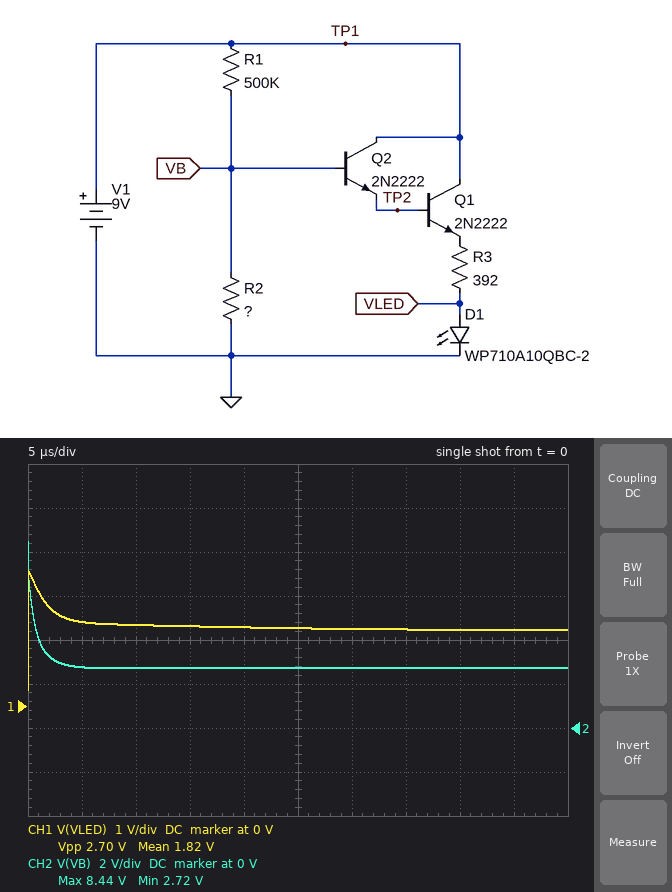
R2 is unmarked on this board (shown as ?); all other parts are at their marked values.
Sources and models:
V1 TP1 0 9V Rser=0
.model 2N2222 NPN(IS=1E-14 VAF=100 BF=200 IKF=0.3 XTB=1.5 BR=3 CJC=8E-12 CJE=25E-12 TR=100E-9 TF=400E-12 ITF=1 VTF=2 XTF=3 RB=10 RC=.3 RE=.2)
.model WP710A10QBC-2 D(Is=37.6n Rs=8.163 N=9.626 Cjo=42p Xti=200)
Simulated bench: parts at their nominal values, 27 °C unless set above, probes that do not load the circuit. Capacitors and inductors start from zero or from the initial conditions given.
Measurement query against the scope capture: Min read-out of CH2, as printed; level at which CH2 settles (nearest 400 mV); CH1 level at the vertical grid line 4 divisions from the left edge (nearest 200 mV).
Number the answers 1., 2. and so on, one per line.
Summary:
1. 2.72 V
2. 2.8 V
3. 1.8 V
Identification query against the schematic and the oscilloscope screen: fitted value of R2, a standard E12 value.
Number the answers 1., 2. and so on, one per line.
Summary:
1. 220 kΩ
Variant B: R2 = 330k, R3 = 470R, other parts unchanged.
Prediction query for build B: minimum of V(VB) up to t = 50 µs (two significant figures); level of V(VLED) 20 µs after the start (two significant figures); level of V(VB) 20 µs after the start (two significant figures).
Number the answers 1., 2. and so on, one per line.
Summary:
1. 3.5 V
2. 2.3 V
3. 3.6 V
